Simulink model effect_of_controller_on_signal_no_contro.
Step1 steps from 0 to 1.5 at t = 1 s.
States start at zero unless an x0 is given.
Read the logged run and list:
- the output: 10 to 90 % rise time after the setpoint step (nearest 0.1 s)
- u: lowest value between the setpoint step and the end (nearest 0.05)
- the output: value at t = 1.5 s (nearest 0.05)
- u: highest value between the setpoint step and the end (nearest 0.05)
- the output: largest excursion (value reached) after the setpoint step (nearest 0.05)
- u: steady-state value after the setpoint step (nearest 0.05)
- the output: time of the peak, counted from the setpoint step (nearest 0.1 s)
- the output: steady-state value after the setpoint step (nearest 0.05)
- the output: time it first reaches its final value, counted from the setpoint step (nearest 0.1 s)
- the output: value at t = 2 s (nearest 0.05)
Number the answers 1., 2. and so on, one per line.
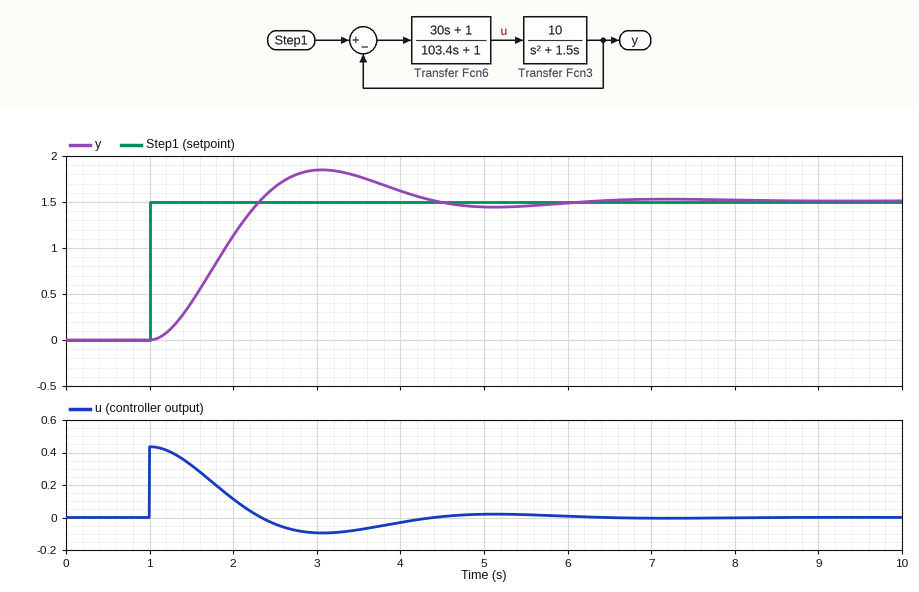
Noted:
1. 0.9 s
2. -0.10
3. 0.40
4. 0.45
5. 1.85
6. 0.00
7. 2.1 s
8. 1.50
9. 1.3 s
10. 1.15
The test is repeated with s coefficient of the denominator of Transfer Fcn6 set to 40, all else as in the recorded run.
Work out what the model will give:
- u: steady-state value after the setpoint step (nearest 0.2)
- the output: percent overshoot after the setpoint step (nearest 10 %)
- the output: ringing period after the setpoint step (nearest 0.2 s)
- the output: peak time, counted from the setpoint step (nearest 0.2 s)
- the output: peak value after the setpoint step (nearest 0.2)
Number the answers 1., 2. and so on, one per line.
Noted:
1. 0.0
2. 40 %
3. 2.4 s
4. 1.2 s
5. 2.2
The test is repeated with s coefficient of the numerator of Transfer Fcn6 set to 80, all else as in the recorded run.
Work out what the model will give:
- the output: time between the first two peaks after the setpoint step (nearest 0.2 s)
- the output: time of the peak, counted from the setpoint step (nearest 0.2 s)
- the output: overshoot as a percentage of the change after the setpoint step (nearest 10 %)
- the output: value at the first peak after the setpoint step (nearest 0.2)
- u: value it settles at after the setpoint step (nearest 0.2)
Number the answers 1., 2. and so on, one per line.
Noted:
1. 2.4 s
2. 1.2 s
3. 40 %
4. 2.2
5. 0.0
